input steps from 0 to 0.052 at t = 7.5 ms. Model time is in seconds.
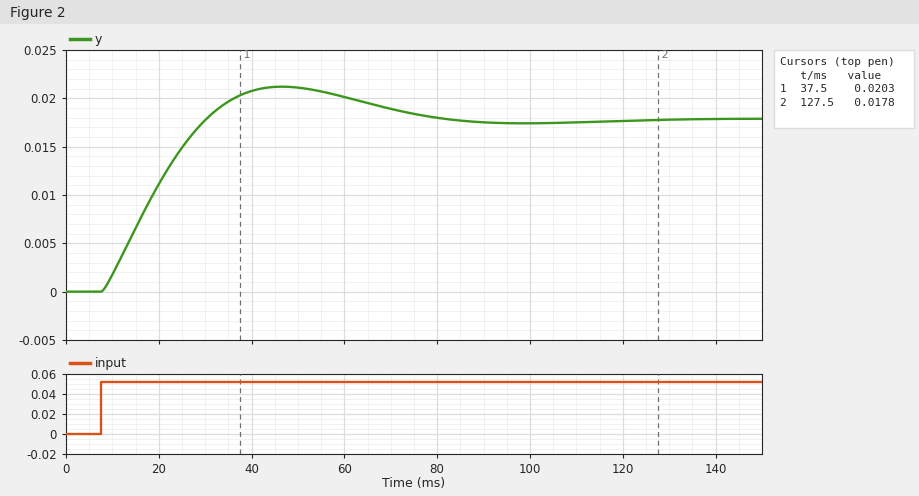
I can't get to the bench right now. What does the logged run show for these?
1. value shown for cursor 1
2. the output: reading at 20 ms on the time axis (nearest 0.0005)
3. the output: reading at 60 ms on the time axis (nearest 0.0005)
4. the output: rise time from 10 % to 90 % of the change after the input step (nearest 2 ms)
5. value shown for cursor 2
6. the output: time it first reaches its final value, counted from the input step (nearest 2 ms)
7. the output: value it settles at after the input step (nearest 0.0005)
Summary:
0.0203
0.0110
0.0200
16 ms
0.0178
22 ms
0.0180
